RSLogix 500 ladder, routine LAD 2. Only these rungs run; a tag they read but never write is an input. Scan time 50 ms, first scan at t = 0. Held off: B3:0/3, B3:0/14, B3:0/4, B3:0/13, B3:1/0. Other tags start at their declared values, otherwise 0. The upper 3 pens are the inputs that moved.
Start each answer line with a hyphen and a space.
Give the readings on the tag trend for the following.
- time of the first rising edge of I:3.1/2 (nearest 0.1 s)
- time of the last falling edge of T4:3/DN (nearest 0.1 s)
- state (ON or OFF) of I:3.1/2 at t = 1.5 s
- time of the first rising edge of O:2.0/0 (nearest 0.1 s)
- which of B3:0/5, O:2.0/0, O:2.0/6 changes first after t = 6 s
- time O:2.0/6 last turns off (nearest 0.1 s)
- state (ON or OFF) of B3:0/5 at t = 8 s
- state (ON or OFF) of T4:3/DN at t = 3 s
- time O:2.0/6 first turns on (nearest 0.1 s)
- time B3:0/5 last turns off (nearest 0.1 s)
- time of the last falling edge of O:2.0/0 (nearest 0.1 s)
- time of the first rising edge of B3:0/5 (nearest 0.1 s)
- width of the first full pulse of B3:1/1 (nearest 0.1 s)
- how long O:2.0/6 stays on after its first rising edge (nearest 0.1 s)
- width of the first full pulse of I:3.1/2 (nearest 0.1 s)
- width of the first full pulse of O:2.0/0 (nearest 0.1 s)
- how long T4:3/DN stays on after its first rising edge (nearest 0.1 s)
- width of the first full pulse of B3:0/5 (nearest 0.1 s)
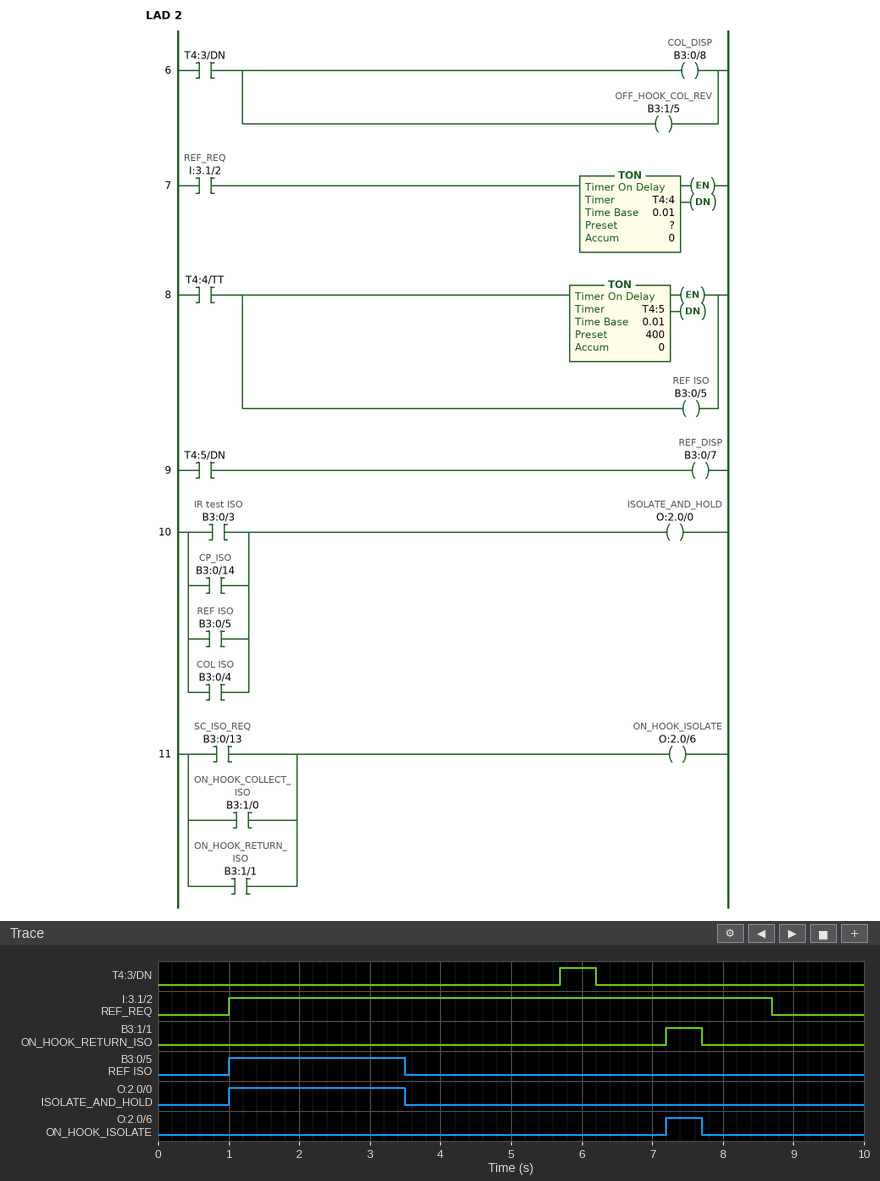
- 1.0 s
- 6.2 s
- ON
- 1.0 s
- O:2.0/6
- 7.7 s
- OFF
- OFF
- 7.2 s
- 3.5 s
- 3.5 s
- 1.0 s
- 0.5 s
- 0.5 s
- 7.7 s
- 2.5 s
- 0.5 s
- 2.5 s
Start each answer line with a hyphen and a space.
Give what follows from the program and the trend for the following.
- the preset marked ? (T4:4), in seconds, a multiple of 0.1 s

- 2.5 s
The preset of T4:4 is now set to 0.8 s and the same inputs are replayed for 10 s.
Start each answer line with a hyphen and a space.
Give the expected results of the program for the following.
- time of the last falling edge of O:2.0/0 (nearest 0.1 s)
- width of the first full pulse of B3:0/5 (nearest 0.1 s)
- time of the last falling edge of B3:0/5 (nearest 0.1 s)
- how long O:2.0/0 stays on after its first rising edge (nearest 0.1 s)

- 1.8 s
- 0.8 s
- 1.8 s
- 0.8 s
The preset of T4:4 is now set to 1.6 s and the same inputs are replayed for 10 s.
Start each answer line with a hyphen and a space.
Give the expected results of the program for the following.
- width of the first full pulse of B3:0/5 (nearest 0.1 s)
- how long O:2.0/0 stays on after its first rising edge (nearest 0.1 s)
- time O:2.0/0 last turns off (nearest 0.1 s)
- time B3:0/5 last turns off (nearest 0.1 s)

- 1.6 s
- 1.6 s
- 2.6 s
- 2.6 s
